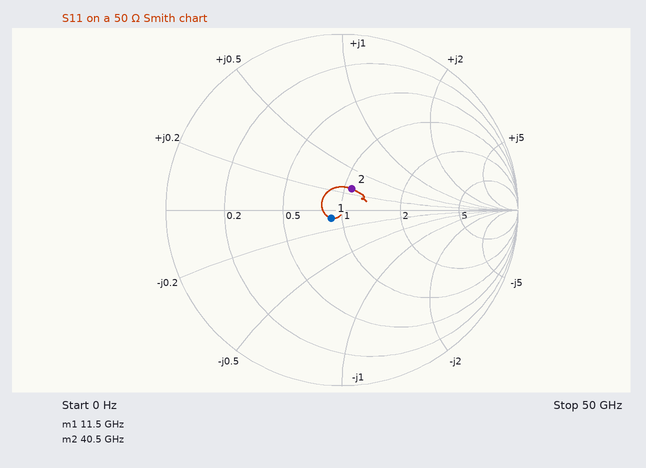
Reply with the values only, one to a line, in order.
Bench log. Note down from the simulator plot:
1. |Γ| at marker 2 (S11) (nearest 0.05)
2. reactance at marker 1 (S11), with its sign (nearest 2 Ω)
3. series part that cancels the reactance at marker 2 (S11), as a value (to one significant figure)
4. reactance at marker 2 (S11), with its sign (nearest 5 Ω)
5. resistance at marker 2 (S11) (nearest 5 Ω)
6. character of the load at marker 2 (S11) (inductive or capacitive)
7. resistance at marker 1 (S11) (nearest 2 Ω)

0.15
-4 Ω
300 fF
+15 Ω
55 Ω
inductive
44 Ω
